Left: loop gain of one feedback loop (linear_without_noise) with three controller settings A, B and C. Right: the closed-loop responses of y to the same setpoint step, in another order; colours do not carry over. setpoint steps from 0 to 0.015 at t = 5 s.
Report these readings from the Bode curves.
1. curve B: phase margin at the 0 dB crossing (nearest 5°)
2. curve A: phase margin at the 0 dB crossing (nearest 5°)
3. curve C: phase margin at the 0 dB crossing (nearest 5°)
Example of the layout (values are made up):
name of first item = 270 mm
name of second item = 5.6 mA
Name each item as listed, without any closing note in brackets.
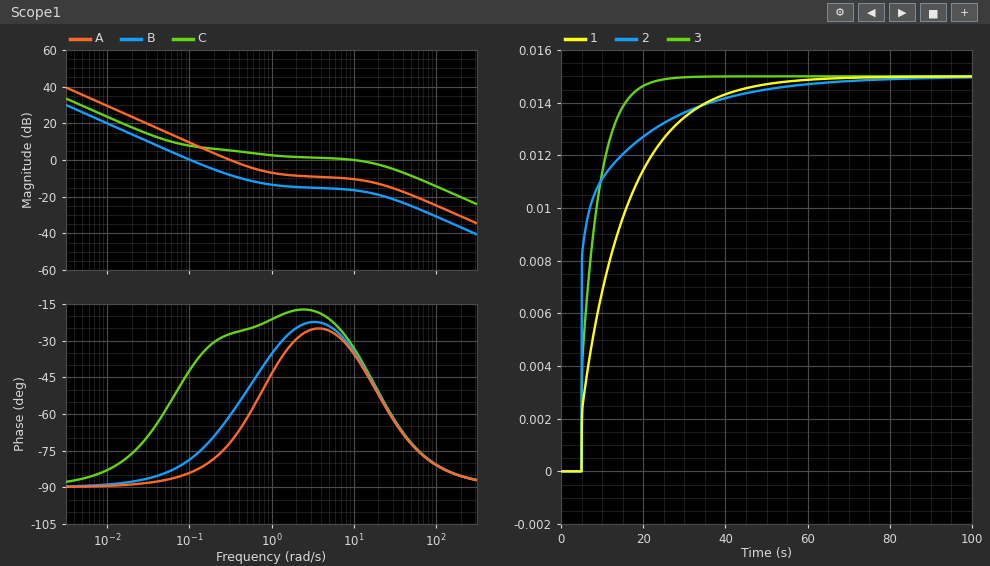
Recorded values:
curve B: phase margin at the 0 dB crossing = 100°
curve A: phase margin at the 0 dB crossing = 110°
curve C: phase margin at the 0 dB crossing = 145°
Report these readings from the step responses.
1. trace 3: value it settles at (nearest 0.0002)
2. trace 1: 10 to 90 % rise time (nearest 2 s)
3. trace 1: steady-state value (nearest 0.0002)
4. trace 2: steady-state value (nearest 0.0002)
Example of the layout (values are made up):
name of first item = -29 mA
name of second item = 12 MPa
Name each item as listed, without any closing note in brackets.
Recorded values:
trace 3: value it settles at = 0.0150
trace 1: 10 to 90 % rise time = 26 s
trace 1: steady-state value = 0.0150
trace 2: steady-state value = 0.0150
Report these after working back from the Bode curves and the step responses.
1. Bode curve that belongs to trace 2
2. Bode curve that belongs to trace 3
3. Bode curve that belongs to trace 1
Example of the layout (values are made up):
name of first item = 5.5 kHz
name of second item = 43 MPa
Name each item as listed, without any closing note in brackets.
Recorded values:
Bode curve that belongs to trace 2 = C
Bode curve that belongs to trace 3 = A
Bode curve that belongs to trace 1 = B
